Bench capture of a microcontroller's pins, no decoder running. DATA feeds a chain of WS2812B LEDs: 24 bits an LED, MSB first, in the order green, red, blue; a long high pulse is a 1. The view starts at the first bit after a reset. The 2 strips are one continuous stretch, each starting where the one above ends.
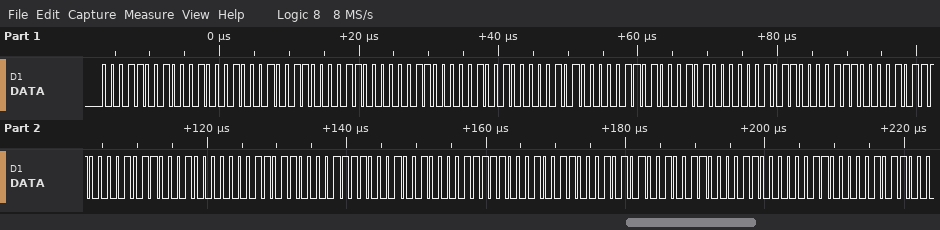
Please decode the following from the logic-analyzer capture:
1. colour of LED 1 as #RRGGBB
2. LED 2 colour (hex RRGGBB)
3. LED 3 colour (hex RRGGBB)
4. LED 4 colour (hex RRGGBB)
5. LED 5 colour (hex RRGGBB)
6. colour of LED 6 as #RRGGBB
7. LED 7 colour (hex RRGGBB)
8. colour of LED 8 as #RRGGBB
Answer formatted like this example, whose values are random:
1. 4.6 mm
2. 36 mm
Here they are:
1. #111913
2. #0C0C12
3. #0D0A14
4. #0E0B17
5. #100B1B
6. #120F1F
7. #151326
8. #18182C
